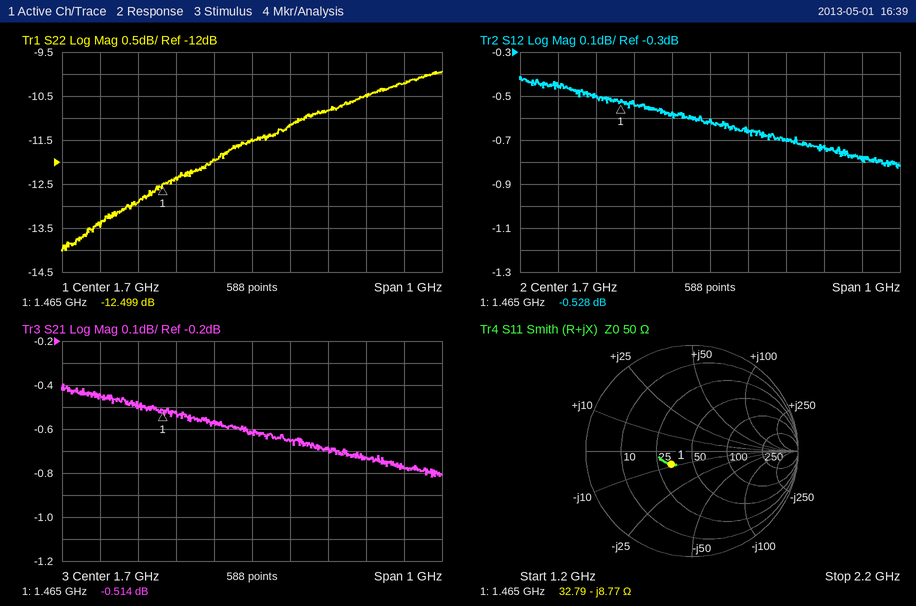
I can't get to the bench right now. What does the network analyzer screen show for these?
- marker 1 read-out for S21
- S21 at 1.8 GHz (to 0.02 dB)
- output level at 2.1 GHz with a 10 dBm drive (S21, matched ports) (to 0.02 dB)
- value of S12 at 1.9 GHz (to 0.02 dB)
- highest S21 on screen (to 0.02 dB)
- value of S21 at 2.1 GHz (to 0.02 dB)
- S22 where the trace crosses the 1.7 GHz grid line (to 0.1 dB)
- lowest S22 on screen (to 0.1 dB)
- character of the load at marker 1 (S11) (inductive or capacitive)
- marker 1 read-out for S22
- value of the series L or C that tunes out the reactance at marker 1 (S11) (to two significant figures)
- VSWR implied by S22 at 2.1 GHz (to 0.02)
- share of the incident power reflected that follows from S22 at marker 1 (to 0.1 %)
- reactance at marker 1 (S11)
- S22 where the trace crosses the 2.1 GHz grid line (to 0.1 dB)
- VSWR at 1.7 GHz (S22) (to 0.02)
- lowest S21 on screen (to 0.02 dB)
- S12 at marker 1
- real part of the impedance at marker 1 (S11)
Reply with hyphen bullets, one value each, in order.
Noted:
- -0.514 dB
- -0.66 dB
- 9.22 dBm
- -0.70 dB
- -0.40 dB
- -0.78 dB
- -11.5 dB
- -14.0 dB
- capacitive
- -12.499 dB
- 950 pH
- 1.90
- 5.6 %
- -8.77 Ω
- -10.2 dB
- 1.72
- -0.82 dB
- -0.528 dB
- 32.79 Ω
